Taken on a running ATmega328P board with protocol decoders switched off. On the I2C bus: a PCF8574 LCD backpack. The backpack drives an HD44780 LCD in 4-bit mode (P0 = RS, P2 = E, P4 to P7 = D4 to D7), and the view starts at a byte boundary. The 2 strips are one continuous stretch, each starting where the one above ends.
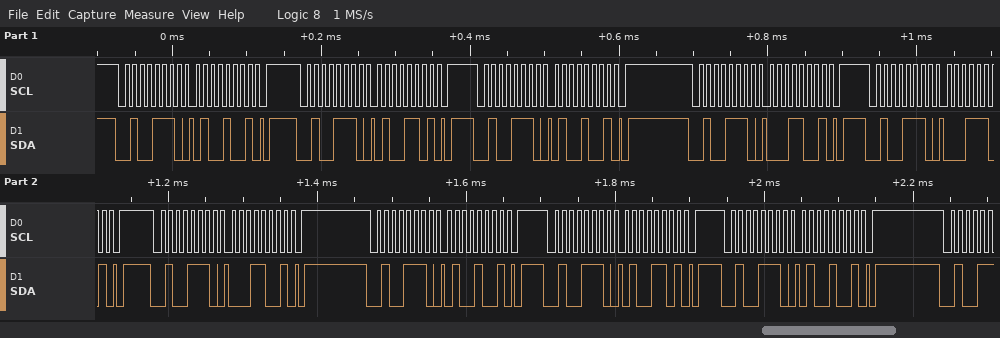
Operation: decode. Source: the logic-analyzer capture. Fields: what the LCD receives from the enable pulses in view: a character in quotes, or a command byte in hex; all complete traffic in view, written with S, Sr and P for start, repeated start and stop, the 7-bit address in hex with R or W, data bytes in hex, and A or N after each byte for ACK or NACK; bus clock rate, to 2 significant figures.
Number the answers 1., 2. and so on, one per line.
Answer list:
1. 'A'
2. S 27W A 49 A P S 27W A 4D A P S 27W A 49 A P S 27W A 19 A P S 27W A 1D A P S 27W A 19 A P S 27W A 49 A P S 27W A 4D A P S 27W A 49 A P
3. 100 kHz
